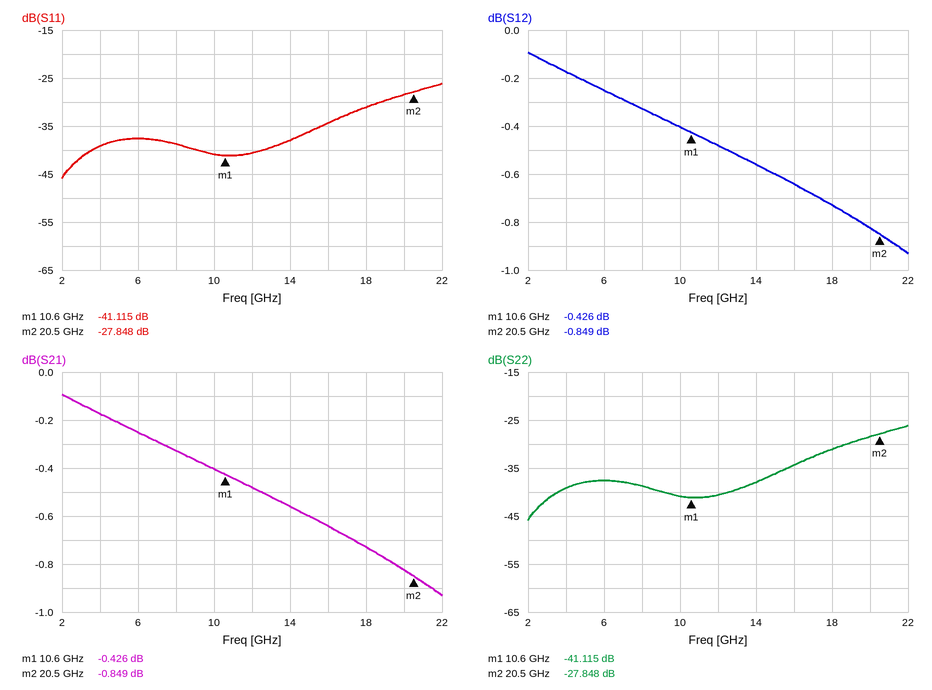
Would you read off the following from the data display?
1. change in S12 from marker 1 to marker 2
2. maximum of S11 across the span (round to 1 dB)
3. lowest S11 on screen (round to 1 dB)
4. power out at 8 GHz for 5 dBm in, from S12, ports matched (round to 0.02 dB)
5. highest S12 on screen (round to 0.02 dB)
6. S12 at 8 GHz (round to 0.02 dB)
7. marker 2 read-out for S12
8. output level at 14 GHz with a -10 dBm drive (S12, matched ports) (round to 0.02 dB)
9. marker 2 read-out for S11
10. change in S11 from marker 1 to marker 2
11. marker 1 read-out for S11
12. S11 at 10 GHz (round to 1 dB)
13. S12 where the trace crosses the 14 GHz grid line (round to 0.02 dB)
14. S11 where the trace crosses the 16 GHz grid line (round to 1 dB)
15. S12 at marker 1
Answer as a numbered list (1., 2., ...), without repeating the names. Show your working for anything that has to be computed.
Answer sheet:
1. -0.849 − (-0.426) = -0.423 dB
2. -26 dB
3. -46 dB
4. 5 dBm + (-0.32 dB) = 4.68 dBm
5. -0.10 dB
6. -0.32 dB
7. -0.849 dB
8. -10 dBm + (-0.56 dB) = -10.56 dBm
9. -27.848 dB
10. -27.848 − (-41.115) = 13.267 dB
11. -41.115 dB
12. -41 dB
13. -0.56 dB
14. -34 dB
15. -0.426 dB
